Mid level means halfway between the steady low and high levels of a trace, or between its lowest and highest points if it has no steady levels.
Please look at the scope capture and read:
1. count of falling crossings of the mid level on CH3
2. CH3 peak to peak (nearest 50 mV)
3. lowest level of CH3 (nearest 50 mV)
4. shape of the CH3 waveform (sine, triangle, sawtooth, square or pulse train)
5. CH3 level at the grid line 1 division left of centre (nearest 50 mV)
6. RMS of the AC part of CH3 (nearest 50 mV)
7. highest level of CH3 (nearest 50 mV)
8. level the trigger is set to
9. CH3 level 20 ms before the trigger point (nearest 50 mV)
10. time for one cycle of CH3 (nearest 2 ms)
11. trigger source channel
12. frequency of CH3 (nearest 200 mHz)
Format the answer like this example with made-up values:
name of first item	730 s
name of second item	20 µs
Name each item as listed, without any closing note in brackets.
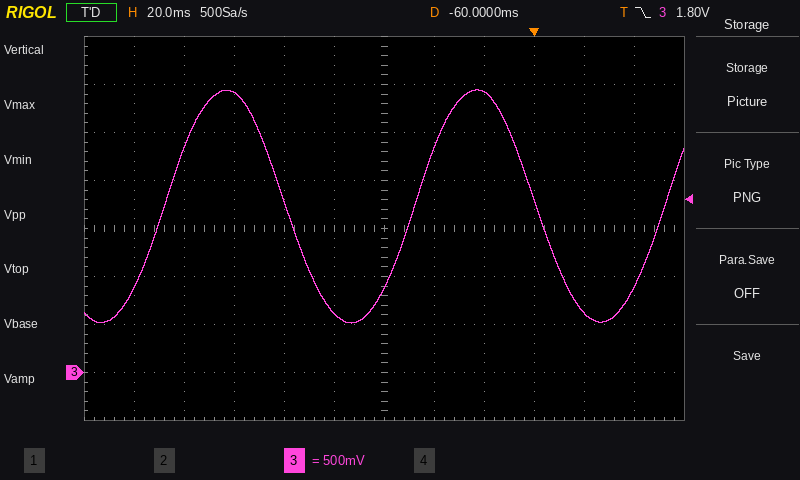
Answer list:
count of falling crossings of the mid level on CH3	2
CH3 peak to peak	2.45 V
lowest level of CH3	500 mV
shape of the CH3 waveform	sine
CH3 level at the grid line 1 division left of centre	600 mV
RMS of the AC part of CH3	850 mV
highest level of CH3	2.95 V
level the trigger is set to	1.80 V
CH3 level 20 ms before the trigger point	2.90 V
time for one cycle of CH3	100 ms
trigger source channel	CH3
frequency of CH3	10.0 Hz
